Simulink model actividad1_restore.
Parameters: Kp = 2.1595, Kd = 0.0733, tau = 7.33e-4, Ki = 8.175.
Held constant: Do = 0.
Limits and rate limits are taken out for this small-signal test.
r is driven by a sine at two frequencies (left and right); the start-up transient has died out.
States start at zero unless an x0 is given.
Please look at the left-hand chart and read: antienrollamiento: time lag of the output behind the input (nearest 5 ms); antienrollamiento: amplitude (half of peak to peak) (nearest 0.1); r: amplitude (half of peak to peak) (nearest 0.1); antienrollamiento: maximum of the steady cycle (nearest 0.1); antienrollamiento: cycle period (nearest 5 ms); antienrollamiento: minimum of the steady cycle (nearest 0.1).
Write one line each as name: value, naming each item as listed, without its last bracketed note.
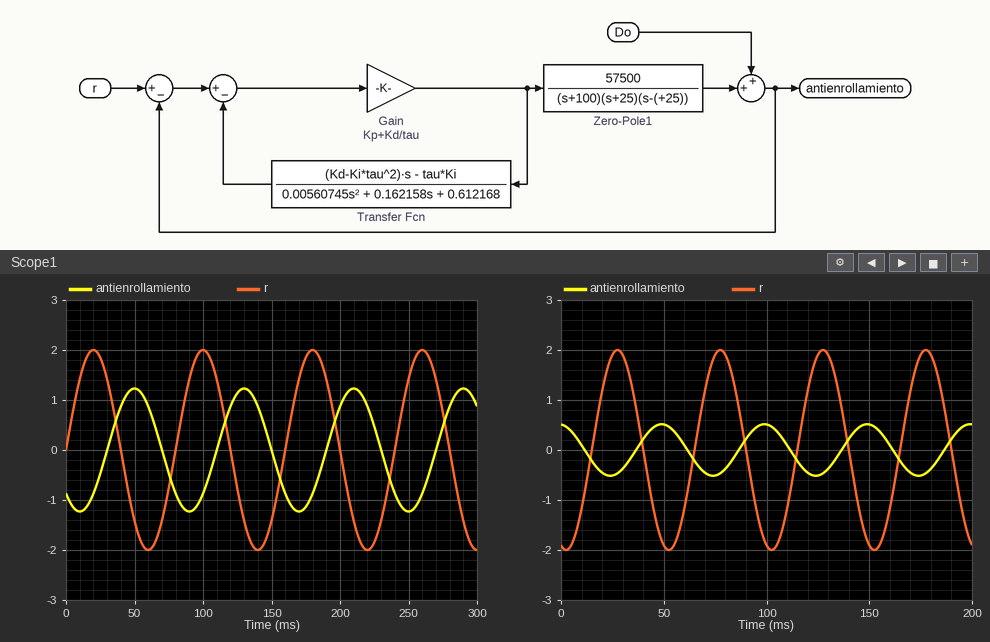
antienrollamiento: time lag of the output behind the input: 30 ms
antienrollamiento: amplitude (half of peak to peak): 1.2
r: amplitude (half of peak to peak): 2.0
antienrollamiento: maximum of the steady cycle: 1.2
antienrollamiento: cycle period: 80 ms
antienrollamiento: minimum of the steady cycle: -1.2
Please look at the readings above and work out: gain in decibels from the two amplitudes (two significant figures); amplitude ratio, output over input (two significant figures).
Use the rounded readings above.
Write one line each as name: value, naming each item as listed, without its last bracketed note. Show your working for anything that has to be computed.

gain in decibels from the two amplitudes: 20 log10(1.2 / 2) = -4.4 dB
amplitude ratio, output over input: 1.2 / 2 = 0.60
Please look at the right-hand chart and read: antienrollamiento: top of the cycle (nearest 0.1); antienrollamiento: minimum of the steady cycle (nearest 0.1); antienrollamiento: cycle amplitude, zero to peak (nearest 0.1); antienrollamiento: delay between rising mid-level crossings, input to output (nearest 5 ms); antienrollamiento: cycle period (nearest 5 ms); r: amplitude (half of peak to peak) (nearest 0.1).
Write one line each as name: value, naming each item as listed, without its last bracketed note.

antienrollamiento: top of the cycle: 0.5
antienrollamiento: minimum of the steady cycle: -0.5
antienrollamiento: cycle amplitude, zero to peak: 0.5
antienrollamiento: delay between rising mid-level crossings, input to output: 20 ms
antienrollamiento: cycle period: 50 ms
r: amplitude (half of peak to peak): 2.0
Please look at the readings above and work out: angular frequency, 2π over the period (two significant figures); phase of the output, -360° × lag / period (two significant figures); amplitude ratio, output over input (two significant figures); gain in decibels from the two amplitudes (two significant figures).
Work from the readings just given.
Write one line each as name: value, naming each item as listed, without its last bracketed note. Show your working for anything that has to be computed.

angular frequency, 2π over the period: 2π / 50 = 0.13 rad/ms
phase of the output, -360° × lag / period: -360 × 20 / 50 = -140°
amplitude ratio, output over input: 0.5 / 2 = 0.25
gain in decibels from the two amplitudes: 20 log10(0.5 / 2) = -12 dB
